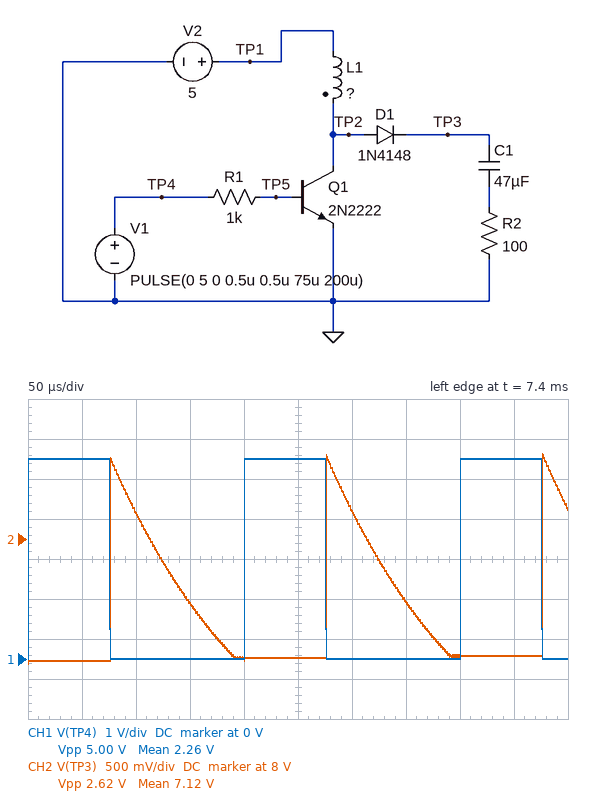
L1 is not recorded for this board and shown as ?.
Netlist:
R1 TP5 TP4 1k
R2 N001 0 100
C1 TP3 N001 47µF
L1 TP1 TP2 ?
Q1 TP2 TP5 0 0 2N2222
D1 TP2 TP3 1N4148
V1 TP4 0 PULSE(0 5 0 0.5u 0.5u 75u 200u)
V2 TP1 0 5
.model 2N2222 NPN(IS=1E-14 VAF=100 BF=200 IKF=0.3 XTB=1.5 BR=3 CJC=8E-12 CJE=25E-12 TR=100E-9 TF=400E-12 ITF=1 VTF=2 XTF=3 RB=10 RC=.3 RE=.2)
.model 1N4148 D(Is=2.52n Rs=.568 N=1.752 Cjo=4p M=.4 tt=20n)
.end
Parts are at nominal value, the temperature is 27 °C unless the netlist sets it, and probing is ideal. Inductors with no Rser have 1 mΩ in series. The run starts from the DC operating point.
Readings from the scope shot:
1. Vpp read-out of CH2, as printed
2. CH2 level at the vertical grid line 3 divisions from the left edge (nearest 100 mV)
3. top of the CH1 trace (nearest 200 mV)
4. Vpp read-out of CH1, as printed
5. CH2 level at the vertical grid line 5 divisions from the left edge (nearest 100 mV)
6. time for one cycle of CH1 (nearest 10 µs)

2.62 V
7.2 V
5.0 V
5.00 V
6.5 V
200 µs
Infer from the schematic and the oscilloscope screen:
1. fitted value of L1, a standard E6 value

15 mH
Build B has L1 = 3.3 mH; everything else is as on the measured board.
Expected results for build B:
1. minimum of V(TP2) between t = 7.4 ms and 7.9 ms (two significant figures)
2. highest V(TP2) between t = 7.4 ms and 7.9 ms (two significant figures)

12 mV
19 V
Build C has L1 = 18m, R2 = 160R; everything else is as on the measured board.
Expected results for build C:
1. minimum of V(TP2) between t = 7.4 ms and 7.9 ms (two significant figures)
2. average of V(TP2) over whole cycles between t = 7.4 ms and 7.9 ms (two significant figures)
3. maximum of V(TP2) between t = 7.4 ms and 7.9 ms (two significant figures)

9.5 mV
5.0 V
10 V
